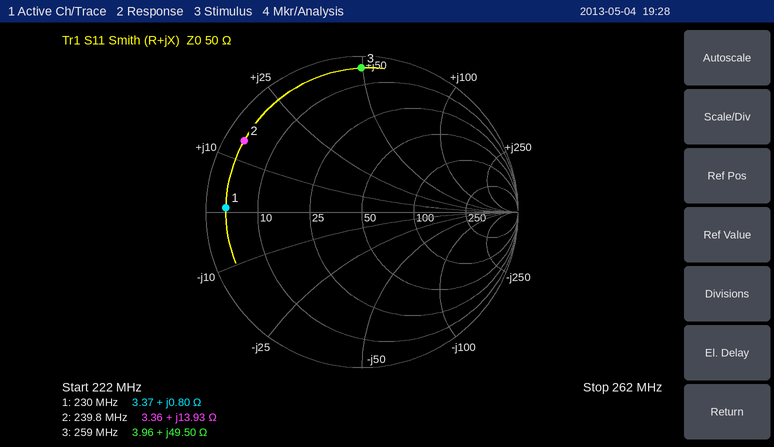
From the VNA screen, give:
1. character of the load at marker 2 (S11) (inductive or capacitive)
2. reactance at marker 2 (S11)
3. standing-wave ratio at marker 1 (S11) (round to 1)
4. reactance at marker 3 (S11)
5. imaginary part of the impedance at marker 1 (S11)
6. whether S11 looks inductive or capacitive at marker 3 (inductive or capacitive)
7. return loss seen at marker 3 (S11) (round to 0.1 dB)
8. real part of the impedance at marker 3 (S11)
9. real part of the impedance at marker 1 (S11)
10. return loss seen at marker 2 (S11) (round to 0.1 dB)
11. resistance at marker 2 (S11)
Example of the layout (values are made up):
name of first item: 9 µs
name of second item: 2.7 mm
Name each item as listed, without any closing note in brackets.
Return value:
character of the load at marker 2 (S11): inductive
reactance at marker 2: +13.93 Ω
standing-wave ratio at marker 1 (S11): 15
reactance at marker 3: +49.50 Ω
imaginary part of the impedance at marker 1: +0.80 Ω
whether S11 looks inductive or capacitive at marker 3: inductive
return loss seen at marker 3 (S11): 0.7 dB
real part of the impedance at marker 3: 3.96 Ω
real part of the impedance at marker 1: 3.37 Ω
return loss seen at marker 2 (S11): 1.1 dB
resistance at marker 2: 3.36 Ω
